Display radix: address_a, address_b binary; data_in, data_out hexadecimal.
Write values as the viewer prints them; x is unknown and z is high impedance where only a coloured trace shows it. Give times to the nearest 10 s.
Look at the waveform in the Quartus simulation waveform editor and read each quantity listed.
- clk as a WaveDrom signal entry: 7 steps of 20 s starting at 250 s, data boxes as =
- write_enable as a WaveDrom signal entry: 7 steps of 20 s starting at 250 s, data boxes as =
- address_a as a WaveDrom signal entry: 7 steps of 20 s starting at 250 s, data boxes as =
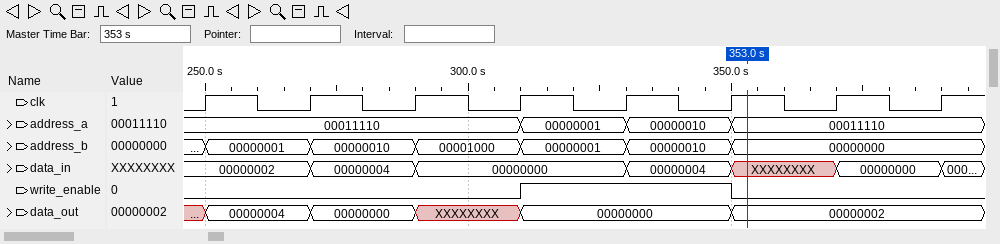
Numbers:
{name: 'clk', wave: 'p......'}
{name: 'write_enable', wave: '0..1.0.'}
{name: 'address_a', wave: '=..===.', data: '00011110 00000001 00000010 00011110'}
